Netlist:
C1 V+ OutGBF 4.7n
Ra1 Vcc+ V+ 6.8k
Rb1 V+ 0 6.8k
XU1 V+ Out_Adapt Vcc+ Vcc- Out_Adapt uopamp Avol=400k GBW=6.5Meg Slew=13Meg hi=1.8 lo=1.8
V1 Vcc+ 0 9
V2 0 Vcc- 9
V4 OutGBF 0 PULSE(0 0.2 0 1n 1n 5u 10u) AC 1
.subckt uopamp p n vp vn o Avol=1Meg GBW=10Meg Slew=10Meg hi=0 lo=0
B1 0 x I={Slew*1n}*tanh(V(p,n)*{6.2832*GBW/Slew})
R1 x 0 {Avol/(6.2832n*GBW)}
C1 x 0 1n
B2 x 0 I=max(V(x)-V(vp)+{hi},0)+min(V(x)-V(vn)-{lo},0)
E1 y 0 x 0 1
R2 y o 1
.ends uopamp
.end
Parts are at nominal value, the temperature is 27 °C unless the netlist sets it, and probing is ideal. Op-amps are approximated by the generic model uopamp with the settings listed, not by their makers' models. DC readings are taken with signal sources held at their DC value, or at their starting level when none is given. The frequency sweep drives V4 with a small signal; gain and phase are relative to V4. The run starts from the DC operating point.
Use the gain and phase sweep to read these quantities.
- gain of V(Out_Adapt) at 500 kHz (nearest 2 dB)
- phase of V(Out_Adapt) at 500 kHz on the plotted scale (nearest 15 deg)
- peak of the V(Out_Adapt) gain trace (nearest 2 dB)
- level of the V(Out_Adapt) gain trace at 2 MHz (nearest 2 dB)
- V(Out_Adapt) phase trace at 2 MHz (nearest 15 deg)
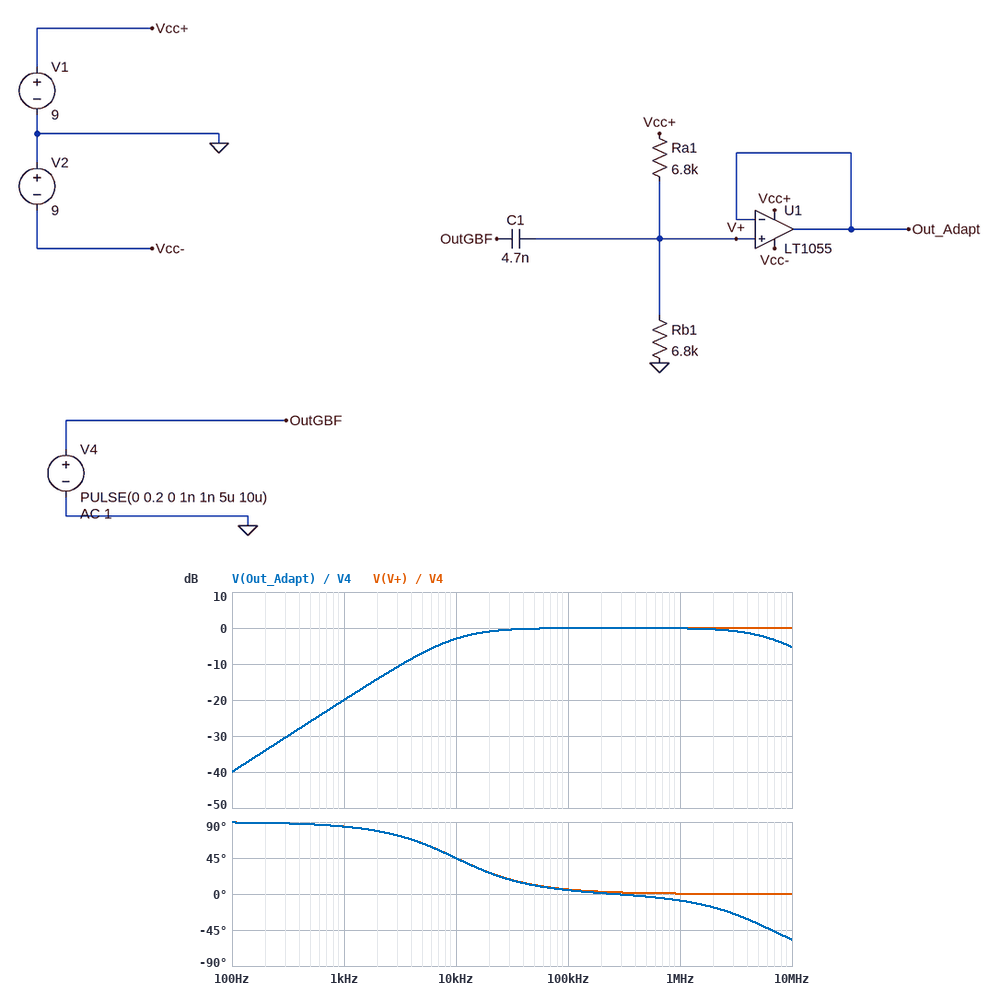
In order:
0 dB
0 deg
0 dB
0 dB
-15 deg
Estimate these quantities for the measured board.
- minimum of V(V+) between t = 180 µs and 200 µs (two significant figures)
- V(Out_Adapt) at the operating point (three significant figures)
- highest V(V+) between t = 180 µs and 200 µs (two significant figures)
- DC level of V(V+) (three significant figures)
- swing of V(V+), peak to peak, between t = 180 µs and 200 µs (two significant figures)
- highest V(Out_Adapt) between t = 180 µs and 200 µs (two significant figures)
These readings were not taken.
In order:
4.4 V
4.50 V
4.6 V
4.50 V
230 mV
4.6 V
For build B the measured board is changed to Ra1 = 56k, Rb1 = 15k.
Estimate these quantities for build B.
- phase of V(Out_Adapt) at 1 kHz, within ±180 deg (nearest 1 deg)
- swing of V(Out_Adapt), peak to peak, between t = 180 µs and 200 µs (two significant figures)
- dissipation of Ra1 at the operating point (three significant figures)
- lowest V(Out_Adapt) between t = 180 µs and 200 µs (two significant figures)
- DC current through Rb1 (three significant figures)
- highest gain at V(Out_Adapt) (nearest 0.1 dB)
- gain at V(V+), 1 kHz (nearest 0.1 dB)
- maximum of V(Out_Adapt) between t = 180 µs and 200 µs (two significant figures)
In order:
71 deg
210 mV
900 µW
1.8 V
127 µA
0 dB
-9.6 dB
2.0 V
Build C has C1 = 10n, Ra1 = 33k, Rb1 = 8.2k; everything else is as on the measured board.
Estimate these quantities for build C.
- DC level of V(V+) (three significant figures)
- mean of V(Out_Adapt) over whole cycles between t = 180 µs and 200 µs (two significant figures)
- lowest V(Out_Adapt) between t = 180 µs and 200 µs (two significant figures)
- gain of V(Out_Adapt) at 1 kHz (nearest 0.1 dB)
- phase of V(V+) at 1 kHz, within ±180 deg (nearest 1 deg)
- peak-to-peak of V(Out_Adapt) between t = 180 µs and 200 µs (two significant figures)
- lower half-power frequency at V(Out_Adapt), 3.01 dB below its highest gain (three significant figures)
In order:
1.79 V
1.8 V
1.7 V
-8.4 dB
68 deg
210 mV
2.42 kHz
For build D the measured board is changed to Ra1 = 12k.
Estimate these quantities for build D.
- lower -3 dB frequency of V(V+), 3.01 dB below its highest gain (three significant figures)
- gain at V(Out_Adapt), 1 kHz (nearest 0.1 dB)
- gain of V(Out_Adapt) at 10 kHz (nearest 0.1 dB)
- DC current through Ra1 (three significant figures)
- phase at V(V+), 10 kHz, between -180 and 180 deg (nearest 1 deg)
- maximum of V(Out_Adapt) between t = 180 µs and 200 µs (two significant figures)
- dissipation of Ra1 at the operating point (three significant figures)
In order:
7.80 kHz
-17.9 dB
-2.1 dB
479 µA
38 deg
3.4 V
2.75 mW
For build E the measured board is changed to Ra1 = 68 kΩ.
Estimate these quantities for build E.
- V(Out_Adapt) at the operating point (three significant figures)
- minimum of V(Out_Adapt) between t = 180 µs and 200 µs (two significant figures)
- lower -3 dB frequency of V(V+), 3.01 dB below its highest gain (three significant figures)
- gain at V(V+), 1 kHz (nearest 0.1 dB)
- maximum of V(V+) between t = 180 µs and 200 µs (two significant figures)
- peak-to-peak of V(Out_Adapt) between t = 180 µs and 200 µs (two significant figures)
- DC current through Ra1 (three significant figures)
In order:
818 mV
710 mV
5.48 kHz
-14.9 dB
930 mV
220 mV
120 µA
